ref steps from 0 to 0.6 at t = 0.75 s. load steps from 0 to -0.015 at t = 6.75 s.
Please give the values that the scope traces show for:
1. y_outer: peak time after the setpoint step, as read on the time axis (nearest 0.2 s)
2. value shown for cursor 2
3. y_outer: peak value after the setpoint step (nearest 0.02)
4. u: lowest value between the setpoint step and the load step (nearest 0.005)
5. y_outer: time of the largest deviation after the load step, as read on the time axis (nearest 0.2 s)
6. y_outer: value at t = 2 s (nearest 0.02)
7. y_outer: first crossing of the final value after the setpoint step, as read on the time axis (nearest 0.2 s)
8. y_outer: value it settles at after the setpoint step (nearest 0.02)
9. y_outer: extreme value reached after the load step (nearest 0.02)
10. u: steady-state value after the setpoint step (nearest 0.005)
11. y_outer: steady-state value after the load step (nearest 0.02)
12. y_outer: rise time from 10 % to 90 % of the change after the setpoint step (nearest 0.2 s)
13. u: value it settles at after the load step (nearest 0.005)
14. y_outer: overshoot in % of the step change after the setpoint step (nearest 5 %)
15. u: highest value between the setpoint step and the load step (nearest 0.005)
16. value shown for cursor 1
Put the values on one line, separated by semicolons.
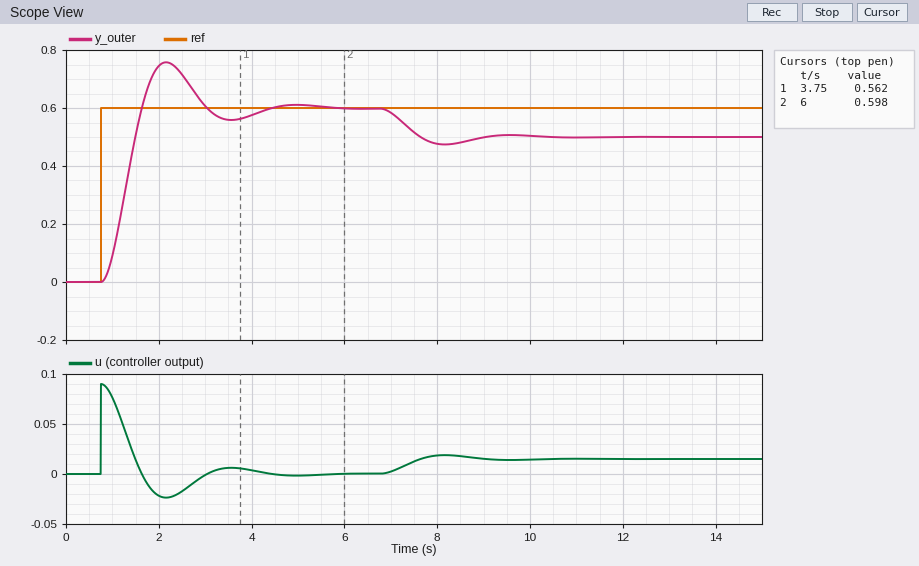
2.2 s; 0.598; 0.76; -0.025; 8.2 s; 0.74; 1.6 s; 0.60; 0.48; 0.000; 0.50; 0.6 s; 0.015; 25 %; 0.090; 0.562
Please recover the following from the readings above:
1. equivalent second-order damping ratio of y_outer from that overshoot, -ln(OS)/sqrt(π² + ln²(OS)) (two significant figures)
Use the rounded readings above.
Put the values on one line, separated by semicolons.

0.40
